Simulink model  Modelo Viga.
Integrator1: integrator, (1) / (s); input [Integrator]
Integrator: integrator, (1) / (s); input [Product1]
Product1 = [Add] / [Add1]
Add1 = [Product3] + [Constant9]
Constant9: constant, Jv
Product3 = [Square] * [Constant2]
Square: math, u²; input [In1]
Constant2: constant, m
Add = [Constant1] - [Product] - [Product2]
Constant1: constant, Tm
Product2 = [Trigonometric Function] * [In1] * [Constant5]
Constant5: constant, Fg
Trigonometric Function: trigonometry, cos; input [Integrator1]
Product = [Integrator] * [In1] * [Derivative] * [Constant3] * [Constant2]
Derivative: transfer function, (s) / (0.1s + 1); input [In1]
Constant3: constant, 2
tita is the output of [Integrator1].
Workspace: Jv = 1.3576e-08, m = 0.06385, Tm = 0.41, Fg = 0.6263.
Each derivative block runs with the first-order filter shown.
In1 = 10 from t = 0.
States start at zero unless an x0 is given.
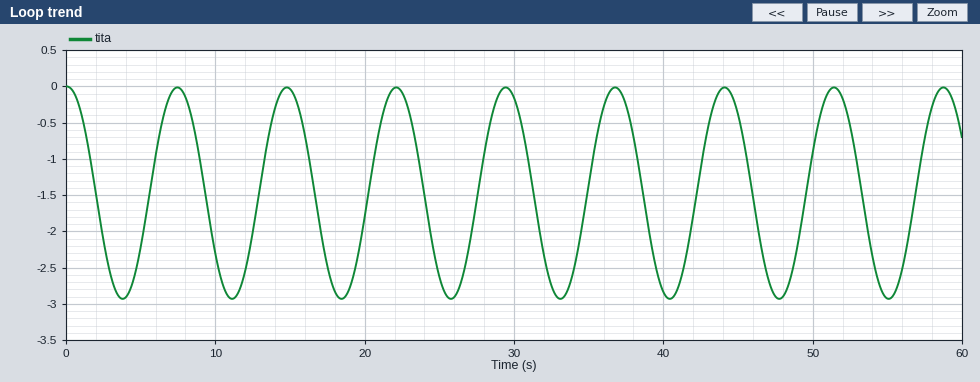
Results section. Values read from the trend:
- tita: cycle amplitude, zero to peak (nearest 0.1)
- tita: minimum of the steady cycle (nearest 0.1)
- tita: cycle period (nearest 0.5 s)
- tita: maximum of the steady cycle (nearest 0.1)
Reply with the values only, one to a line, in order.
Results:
1.5
-2.9
7.5 s
0.0
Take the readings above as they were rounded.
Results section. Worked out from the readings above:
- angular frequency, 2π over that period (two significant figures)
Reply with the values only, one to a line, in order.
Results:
0.84 rad/s
